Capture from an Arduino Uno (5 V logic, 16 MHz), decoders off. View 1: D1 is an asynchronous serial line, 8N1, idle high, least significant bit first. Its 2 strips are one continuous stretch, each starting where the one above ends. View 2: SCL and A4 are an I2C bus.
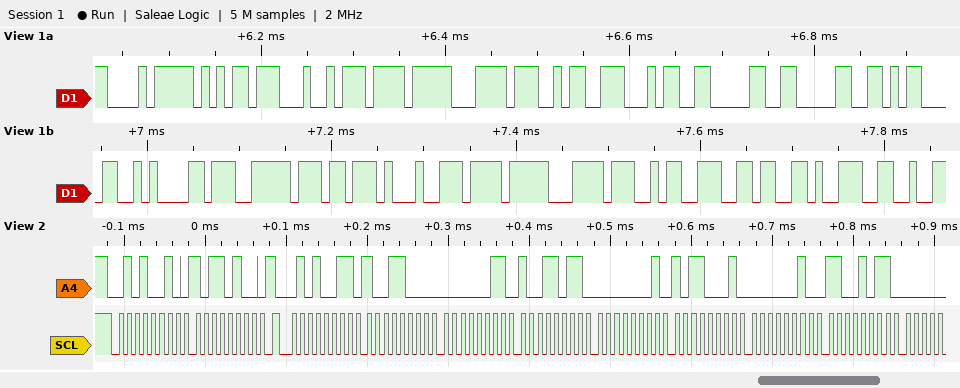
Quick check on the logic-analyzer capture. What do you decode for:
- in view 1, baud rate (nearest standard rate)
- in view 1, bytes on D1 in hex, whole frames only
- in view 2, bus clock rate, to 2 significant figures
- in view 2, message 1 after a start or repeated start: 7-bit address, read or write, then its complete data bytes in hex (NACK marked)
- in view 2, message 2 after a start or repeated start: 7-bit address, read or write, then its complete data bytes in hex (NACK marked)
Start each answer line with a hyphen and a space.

- 115200 baud
- E8 B5 A4 EF BC 9A 34 30 30 0D 0A E7 B7 91 EF BC 9A 36 39
- 100 kHz
- 0x29 write: B4
- 0x29 read: 98 03 9B 01 B1 02 CB
